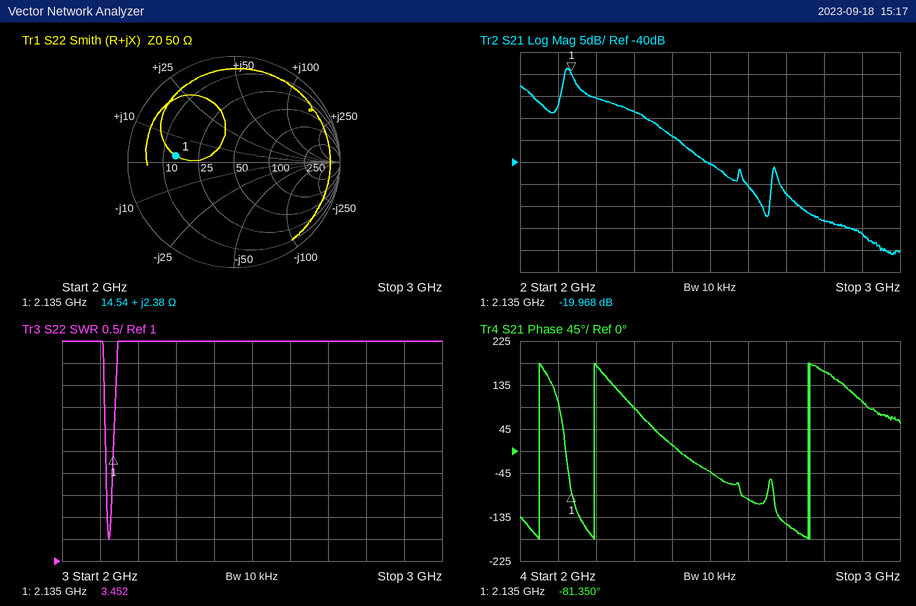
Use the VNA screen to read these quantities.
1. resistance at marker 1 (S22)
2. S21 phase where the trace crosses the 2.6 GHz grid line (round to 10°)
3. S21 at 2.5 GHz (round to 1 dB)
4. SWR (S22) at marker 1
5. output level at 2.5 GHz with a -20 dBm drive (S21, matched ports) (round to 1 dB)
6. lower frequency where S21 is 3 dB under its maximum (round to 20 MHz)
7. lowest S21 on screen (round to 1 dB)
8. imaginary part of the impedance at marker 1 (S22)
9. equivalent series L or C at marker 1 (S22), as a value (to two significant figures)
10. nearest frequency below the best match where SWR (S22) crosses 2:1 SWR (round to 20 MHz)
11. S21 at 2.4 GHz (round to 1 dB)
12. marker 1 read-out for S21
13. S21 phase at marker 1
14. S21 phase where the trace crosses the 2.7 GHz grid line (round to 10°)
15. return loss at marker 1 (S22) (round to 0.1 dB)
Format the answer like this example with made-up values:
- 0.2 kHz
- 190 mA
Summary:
- 14.54 Ω
- -100°
- -40 dB
- 3.452
- -60 dBm
- 2.12 GHz
- -61 dB
- +2.38 Ω
- 180 pH
- 2.12 GHz
- -34 dB
- -19.968 dB
- -81.350°
- -150°
- 5.2 dB
